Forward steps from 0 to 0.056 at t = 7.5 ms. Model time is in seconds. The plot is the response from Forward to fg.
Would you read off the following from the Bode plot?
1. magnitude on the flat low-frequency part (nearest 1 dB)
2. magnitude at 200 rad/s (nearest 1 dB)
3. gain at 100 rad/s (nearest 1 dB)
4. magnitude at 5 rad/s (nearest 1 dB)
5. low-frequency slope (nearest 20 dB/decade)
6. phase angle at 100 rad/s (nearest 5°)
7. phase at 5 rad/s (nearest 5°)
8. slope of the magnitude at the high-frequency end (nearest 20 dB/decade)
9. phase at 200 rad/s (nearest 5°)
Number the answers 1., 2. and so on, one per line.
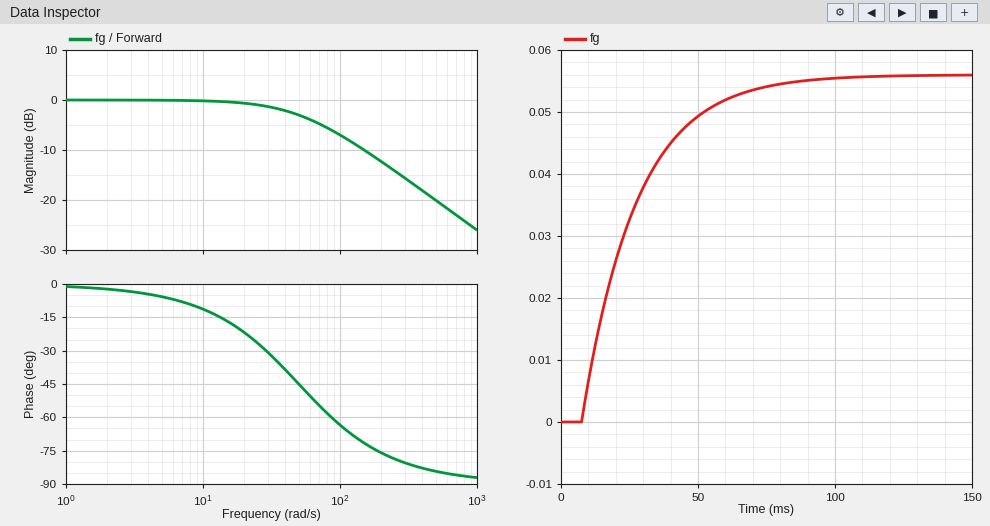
1. 0 dB
2. -12 dB
3. -7 dB
4. 0 dB
5. 0 dB/decade
6. -65°
7. -5°
8. -20 dB/decade
9. -75°
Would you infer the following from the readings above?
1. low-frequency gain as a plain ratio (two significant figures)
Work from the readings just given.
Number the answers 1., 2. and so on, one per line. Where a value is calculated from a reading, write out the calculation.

1. 10^(0 / 20) = 1.0
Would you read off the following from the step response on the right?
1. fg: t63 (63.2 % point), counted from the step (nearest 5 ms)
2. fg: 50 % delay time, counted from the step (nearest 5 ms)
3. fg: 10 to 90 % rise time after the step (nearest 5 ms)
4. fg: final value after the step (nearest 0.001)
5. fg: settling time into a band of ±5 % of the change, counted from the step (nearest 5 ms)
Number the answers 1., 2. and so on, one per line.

1. 20 ms
2. 15 ms
3. 45 ms
4. 0.056
5. 60 ms
